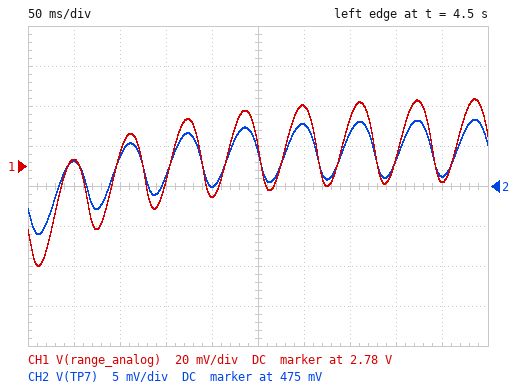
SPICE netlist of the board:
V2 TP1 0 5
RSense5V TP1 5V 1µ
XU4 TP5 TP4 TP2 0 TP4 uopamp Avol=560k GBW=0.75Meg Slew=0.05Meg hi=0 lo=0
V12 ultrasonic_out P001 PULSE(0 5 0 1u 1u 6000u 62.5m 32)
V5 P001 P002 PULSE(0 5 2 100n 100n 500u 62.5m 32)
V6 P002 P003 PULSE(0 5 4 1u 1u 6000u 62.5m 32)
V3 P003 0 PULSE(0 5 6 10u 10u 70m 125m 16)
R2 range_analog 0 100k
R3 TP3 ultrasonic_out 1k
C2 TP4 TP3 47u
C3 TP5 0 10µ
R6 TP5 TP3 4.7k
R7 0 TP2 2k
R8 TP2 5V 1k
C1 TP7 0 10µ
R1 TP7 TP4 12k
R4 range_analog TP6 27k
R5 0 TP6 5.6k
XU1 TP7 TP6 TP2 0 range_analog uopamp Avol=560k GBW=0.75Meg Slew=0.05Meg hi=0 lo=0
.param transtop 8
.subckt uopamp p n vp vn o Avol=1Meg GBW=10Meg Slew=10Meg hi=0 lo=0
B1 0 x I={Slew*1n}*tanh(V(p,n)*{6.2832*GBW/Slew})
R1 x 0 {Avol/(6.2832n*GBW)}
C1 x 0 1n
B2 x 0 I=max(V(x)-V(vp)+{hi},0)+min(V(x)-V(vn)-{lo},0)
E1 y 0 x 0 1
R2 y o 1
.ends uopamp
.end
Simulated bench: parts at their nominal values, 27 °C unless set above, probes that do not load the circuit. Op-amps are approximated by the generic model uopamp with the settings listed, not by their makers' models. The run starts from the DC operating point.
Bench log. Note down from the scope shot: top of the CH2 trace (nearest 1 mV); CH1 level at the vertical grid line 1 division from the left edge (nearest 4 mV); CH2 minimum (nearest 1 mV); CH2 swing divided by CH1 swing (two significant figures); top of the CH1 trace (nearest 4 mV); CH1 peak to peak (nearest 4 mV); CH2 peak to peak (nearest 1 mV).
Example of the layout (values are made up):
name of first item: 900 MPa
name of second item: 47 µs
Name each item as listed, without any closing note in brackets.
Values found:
top of the CH2 trace: 483 mV
CH1 level at the vertical grid line 1 division from the left edge: 2.784 V
CH2 minimum: 469 mV
CH2 swing divided by CH1 swing: 0.17
top of the CH1 trace: 2.812 V
CH1 peak to peak: 84 mV
CH2 peak to peak: 14 mV
